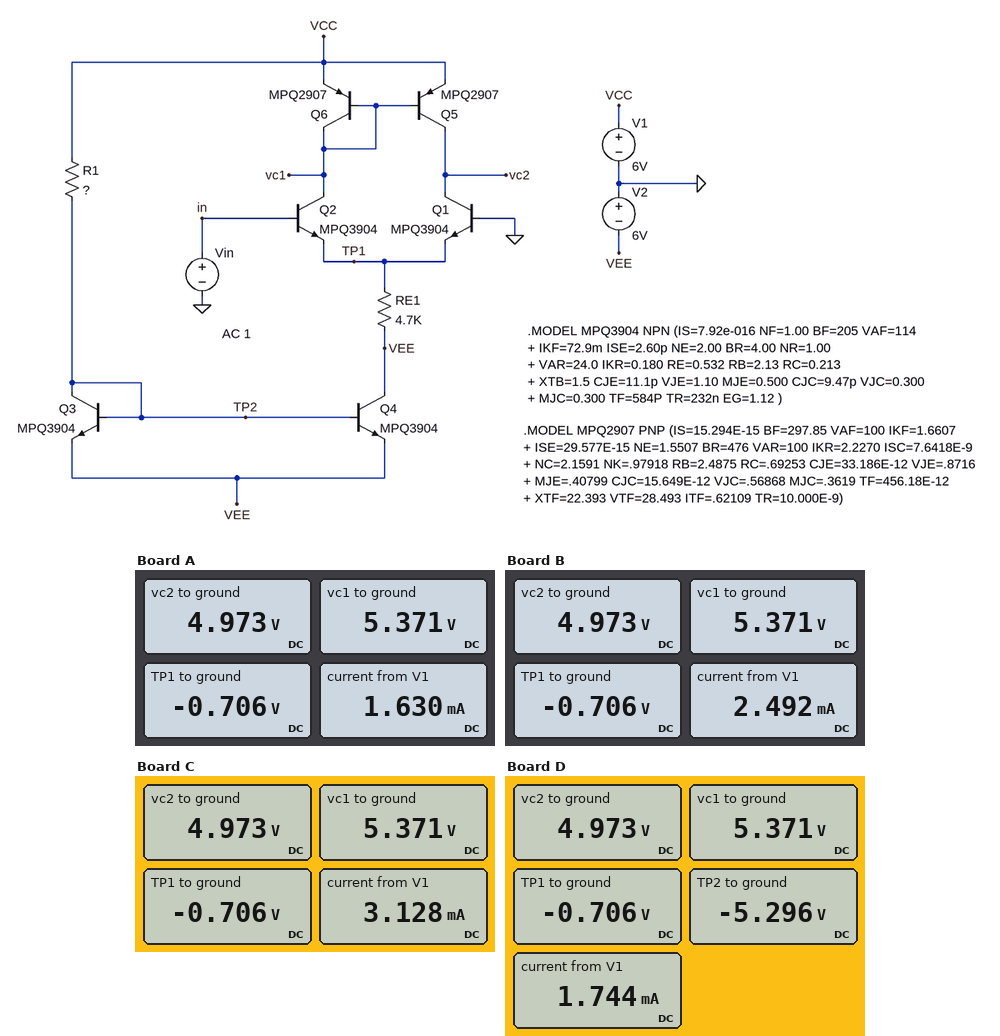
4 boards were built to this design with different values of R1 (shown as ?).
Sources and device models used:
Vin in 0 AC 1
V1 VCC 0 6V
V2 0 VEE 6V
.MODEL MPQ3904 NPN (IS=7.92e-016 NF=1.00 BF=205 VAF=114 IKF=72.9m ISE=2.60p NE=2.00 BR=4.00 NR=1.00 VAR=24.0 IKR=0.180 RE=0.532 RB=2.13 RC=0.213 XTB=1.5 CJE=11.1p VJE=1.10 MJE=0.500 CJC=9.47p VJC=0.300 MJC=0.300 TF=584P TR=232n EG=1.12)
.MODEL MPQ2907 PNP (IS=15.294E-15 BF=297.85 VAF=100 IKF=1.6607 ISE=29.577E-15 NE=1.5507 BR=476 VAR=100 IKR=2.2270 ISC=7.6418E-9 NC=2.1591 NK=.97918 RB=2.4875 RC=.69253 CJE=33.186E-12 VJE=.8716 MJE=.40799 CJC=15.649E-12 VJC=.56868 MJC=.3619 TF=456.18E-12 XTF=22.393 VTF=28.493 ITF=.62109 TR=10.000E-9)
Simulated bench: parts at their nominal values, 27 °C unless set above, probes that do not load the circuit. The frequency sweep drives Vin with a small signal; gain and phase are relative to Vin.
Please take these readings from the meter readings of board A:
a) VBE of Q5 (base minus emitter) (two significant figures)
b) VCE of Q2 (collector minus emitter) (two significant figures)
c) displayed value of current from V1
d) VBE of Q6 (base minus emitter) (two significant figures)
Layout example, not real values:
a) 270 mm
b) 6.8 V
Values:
a) -630 mV
b) 6.1 V
c) 1.630 mA
d) -630 mV
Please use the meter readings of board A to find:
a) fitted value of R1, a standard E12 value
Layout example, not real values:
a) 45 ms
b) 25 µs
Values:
a) 22 kΩ
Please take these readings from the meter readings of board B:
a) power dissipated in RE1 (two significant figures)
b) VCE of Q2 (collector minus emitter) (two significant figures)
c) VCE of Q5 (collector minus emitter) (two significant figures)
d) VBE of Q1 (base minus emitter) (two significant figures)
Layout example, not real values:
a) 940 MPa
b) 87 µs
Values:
a) 6.0 mW
b) 6.1 V
c) -1.0 V
d) 710 mV
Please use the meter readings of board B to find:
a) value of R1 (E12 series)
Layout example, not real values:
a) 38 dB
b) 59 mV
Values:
a) 8.2 kΩ
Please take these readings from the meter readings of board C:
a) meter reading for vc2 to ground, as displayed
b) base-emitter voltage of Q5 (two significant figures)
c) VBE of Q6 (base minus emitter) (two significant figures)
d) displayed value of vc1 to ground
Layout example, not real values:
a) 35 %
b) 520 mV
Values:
a) 4.973 V
b) -630 mV
c) -630 mV
d) 5.371 V
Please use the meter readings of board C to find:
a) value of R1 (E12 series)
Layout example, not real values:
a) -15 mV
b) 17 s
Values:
a) 5.6 kΩ
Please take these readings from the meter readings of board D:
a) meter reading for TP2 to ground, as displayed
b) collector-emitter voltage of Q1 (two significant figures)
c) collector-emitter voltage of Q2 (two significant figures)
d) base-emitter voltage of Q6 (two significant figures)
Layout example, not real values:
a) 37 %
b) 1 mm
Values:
a) -5.296 V
b) 5.7 V
c) 6.1 V
d) -630 mV
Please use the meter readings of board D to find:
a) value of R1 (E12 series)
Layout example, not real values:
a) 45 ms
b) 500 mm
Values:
a) 18 kΩ
